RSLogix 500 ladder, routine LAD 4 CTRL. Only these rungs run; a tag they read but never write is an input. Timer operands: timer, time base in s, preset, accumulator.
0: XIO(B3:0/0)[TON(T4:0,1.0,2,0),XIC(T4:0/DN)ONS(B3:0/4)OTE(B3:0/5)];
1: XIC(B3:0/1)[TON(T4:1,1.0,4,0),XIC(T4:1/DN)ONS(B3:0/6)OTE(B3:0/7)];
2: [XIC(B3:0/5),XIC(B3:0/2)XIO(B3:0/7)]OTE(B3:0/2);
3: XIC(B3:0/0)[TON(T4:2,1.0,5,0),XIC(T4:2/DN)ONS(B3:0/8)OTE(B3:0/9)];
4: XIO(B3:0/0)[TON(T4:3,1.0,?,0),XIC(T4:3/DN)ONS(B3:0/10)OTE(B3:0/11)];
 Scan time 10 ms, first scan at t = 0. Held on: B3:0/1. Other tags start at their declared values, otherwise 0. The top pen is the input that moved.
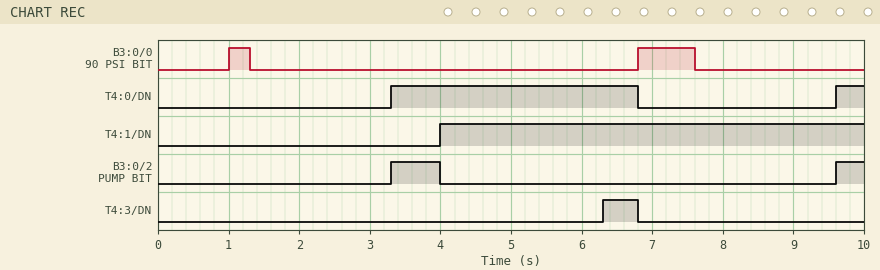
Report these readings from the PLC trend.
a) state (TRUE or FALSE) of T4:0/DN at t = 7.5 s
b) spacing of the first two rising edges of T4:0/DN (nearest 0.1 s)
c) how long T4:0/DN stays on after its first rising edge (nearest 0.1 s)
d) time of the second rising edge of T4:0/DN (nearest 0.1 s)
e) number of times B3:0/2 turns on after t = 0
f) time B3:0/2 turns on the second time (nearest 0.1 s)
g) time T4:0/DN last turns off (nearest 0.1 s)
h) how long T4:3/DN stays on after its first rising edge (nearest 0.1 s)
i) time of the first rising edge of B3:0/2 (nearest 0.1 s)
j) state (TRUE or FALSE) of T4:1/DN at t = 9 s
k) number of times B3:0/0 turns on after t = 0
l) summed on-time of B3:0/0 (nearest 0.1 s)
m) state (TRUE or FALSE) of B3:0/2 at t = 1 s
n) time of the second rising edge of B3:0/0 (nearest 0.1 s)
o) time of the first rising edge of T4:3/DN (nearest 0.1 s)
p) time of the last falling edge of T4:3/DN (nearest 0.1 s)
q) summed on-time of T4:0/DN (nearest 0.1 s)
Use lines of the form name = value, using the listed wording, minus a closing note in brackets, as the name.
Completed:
state (TRUE or FALSE) of T4:0/DN at t = 7.5 s = FALSE
spacing of the first two rising edges of T4:0/DN = 6.3 s
how long T4:0/DN stays on after its first rising edge = 3.5 s
time of the second rising edge of T4:0/DN = 9.6 s
number of times B3:0/2 turns on after t = 0 = 2
time B3:0/2 turns on the second time = 9.6 s
time T4:0/DN last turns off = 6.8 s
how long T4:3/DN stays on after its first rising edge = 0.5 s
time of the first rising edge of B3:0/2 = 3.3 s
state (TRUE or FALSE) of T4:1/DN at t = 9 s = TRUE
number of times B3:0/0 turns on after t = 0 = 2
summed on-time of B3:0/0 = 1.1 s
state (TRUE or FALSE) of B3:0/2 at t = 1 s = FALSE
time of the second rising edge of B3:0/0 = 6.8 s
time of the first rising edge of T4:3/DN = 6.3 s
time of the last falling edge of T4:3/DN = 6.8 s
summed on-time of T4:0/DN = 3.9 s
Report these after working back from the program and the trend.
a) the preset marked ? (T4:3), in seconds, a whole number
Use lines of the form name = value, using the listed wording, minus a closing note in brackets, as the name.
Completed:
the preset marked ? (T4:3), in seconds, a whole number = 5 s
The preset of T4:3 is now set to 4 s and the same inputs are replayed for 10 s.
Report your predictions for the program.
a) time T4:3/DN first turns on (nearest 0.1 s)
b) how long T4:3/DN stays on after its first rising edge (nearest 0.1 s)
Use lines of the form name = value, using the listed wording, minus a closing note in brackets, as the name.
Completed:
time T4:3/DN first turns on = 5.3 s
how long T4:3/DN stays on after its first rising edge = 1.5 s
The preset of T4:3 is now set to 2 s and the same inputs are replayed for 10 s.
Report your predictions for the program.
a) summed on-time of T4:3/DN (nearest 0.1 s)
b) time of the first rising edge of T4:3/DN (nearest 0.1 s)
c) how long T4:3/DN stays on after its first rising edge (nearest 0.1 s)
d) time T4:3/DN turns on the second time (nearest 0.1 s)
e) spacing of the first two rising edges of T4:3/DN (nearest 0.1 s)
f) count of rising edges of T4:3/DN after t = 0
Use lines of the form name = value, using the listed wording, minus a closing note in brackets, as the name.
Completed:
summed on-time of T4:3/DN = 3.9 s
time of the first rising edge of T4:3/DN = 3.3 s
how long T4:3/DN stays on after its first rising edge = 3.5 s
time T4:3/DN turns on the second time = 9.6 s
spacing of the first two rising edges of T4:3/DN = 6.3 s
count of rising edges of T4:3/DN after t = 0 = 2
